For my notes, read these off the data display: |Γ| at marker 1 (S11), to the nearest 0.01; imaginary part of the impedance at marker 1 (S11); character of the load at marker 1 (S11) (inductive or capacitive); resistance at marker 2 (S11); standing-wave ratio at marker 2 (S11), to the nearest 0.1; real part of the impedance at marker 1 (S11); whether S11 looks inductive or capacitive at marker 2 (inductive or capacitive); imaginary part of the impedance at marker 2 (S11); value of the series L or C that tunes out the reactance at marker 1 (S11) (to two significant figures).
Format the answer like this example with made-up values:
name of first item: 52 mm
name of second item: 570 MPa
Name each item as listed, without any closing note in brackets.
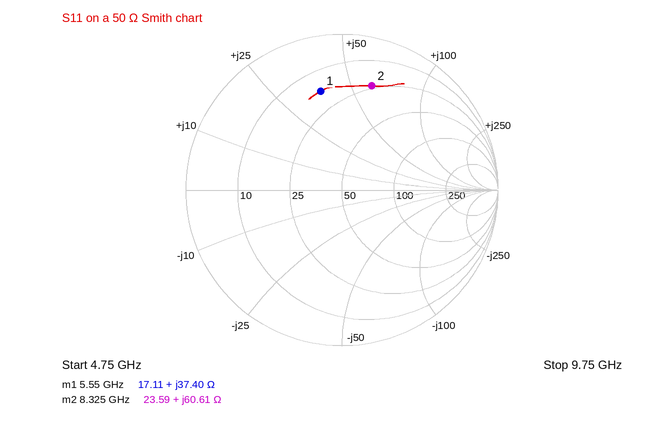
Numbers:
|Γ| at marker 1 (S11), to the nearest 0.01: 0.65
imaginary part of the impedance at marker 1: +37.40 Ω
character of the load at marker 1 (S11): inductive
resistance at marker 2: 23.59 Ω
standing-wave ratio at marker 2 (S11), to the nearest 0.1: 5.5
real part of the impedance at marker 1: 17.11 Ω
whether S11 looks inductive or capacitive at marker 2: inductive
imaginary part of the impedance at marker 2: +60.61 Ω
value of the series L or C that tunes out the reactance at marker 1 (S11): 770 fF
